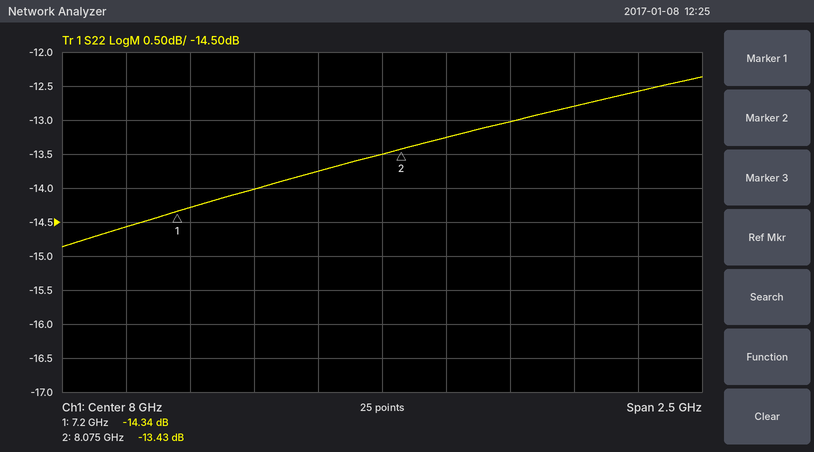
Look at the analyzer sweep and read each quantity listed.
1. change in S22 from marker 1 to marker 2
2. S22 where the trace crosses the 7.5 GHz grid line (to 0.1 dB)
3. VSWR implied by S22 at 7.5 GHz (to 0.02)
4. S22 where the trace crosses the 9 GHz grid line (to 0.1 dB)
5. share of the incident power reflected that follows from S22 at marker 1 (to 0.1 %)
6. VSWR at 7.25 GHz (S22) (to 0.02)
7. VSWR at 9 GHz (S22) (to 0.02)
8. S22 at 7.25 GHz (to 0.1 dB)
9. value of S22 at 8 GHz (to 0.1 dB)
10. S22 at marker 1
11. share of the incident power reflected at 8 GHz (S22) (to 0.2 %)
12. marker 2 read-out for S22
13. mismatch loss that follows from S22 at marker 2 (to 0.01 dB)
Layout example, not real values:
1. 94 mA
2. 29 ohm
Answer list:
1. 0.91 dB
2. -14.0 dB
3. 1.50
4. -12.6 dB
5. 3.7 %
6. 1.48
7. 1.62
8. -14.3 dB
9. -13.5 dB
10. -14.34 dB
11. 4.4 %
12. -13.43 dB
13. 0.20 dB
